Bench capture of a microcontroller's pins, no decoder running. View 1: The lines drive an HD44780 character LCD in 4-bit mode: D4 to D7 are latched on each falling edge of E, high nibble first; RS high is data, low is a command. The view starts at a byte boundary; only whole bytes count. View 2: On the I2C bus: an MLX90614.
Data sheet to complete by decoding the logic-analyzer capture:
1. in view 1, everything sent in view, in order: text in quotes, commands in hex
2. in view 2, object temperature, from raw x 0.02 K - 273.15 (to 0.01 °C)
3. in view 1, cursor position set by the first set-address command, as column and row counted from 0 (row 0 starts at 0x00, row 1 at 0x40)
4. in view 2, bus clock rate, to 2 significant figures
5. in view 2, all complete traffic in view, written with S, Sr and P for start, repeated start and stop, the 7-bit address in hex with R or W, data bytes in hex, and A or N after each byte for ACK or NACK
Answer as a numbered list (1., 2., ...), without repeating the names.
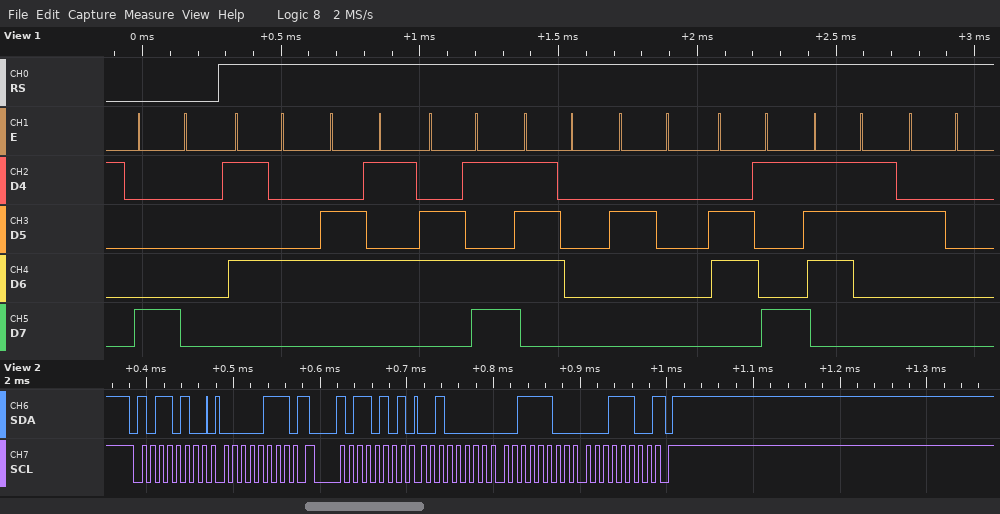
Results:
1. 0x80 "Temp is "
2. 34.69 °C
3. column 0, row 0
4. 100 kHz
5. S 5AW A 07 A Sr 5AR A 20 A 3C A 1C N P
